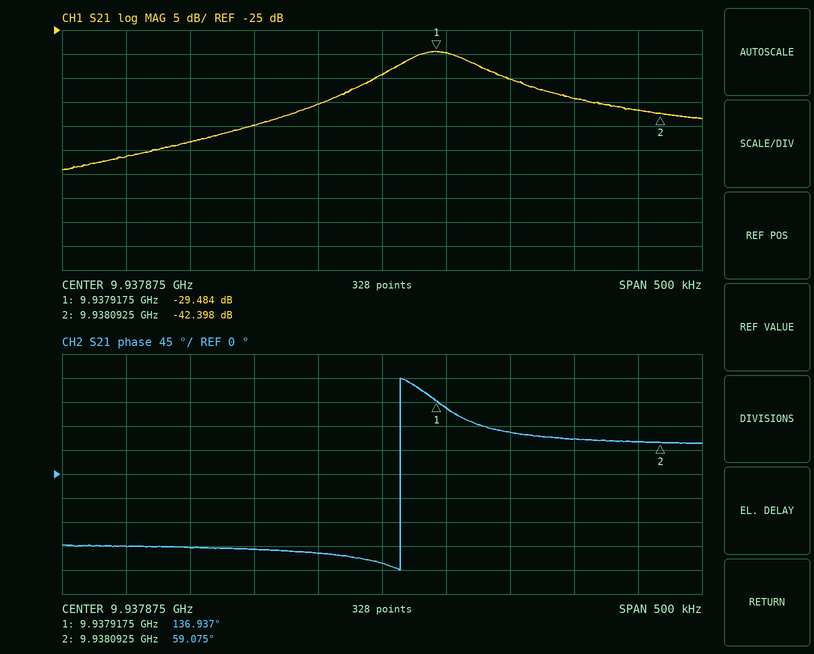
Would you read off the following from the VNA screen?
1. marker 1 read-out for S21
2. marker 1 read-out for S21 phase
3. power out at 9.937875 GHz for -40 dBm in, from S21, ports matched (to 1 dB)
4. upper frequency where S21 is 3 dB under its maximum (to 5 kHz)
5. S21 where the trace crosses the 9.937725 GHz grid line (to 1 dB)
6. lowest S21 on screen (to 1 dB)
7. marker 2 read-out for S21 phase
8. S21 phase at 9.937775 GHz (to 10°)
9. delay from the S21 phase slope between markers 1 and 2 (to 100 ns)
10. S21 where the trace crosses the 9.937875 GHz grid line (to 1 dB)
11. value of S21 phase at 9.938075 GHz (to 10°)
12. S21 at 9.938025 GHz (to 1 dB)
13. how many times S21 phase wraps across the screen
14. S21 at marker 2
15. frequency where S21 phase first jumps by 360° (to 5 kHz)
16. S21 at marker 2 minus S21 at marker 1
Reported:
-29.484 dB
136.937°
-74 dBm
9.937950 GHz
-48 dB
-54 dB
59.075°
-140°
1.2 µs
-34 dB
60°
-39 dB
1
-42.398 dB
9.937890 GHz
-12.914 dB
